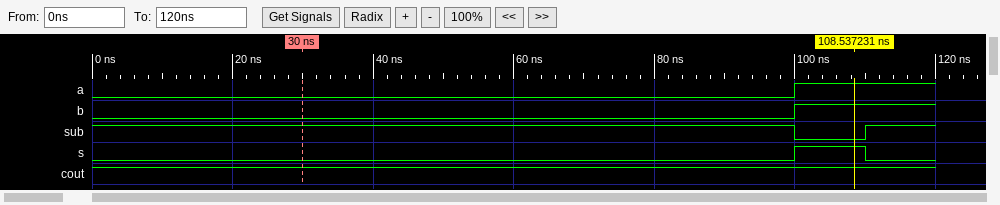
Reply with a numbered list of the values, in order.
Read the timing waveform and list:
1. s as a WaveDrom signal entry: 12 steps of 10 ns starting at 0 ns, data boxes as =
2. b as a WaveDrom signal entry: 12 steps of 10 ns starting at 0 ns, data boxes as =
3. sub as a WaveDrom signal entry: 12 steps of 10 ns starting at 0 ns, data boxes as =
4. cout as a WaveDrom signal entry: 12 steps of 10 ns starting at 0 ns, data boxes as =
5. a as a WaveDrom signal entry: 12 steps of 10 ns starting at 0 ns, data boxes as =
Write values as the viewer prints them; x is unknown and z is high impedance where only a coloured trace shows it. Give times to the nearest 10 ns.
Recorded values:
1. {name: 's', wave: '0.........10'}
2. {name: 'b', wave: '0.........1.'}
3. {name: 'sub', wave: '1.........01'}
4. {name: 'cout', wave: '1...........'}
5. {name: 'a', wave: '0.........1.'}
